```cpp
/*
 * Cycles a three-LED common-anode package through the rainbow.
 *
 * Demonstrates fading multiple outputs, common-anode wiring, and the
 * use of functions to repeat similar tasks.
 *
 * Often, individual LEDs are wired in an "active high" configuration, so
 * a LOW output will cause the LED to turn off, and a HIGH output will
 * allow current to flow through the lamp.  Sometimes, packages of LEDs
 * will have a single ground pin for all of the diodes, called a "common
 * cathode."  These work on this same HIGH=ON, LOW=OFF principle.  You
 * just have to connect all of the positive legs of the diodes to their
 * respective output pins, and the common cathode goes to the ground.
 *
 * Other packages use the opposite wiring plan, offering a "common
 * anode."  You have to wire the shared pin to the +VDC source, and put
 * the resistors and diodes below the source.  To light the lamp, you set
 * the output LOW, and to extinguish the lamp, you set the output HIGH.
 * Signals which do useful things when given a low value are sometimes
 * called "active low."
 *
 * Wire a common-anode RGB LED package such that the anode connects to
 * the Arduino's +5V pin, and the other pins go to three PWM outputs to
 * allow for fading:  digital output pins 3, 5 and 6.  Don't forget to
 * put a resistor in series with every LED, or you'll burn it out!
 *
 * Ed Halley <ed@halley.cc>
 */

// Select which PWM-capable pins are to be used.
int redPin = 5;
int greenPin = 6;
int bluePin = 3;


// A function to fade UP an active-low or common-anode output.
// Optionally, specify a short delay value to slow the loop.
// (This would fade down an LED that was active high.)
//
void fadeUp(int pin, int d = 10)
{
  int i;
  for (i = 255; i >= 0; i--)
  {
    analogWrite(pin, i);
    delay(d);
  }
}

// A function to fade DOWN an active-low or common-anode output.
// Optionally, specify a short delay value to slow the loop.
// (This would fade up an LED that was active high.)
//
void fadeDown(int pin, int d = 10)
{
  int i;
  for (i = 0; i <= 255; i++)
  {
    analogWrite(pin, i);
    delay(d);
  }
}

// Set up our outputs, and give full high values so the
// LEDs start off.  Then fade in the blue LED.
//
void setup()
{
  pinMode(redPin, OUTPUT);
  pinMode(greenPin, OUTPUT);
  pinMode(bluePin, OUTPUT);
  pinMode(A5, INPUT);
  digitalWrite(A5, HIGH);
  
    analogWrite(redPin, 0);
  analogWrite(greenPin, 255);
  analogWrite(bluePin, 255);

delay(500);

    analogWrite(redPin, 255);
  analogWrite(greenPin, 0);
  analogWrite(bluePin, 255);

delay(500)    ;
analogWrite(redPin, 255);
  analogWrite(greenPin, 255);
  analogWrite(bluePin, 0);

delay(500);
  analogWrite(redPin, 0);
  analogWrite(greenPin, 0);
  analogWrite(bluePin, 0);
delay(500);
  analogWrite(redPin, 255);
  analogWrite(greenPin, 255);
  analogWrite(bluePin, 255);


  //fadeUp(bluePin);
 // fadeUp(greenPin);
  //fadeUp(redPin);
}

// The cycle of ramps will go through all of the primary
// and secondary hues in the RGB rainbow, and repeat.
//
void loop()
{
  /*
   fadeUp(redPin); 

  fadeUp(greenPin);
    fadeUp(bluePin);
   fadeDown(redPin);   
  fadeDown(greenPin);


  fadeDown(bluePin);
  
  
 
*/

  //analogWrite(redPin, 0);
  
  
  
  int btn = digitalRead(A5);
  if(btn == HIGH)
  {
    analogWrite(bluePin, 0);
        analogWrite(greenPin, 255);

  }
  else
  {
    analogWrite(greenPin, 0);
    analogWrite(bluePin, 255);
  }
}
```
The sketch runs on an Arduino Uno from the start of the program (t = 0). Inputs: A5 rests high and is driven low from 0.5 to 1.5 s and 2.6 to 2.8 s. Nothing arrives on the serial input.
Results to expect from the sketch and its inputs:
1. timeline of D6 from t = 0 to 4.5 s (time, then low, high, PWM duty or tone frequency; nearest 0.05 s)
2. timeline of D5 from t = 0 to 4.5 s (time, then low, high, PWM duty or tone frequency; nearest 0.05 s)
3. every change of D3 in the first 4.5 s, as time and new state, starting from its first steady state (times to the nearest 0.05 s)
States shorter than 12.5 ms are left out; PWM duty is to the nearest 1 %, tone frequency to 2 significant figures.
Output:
0 s high; 0.5 s low; 1 s high; 1.5 s low; 2 s high; 2.6 s low; 2.8 s high
0 s low; 0.5 s high; 1.5 s low; 2 s high
0 s high; 1 s low; 2.6 s high; 2.8 s low
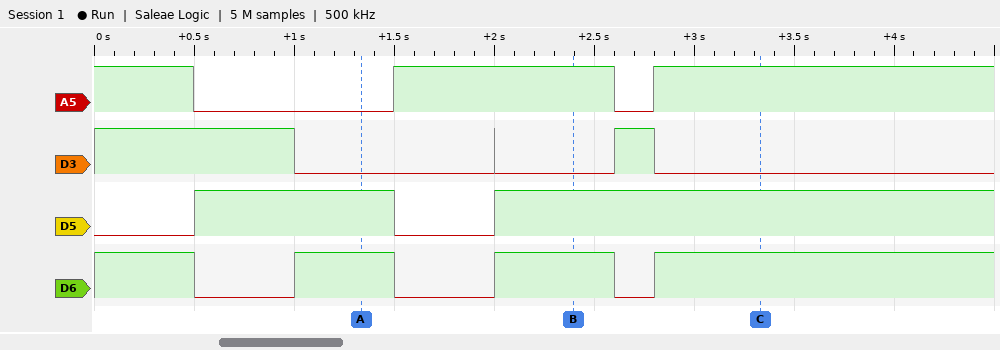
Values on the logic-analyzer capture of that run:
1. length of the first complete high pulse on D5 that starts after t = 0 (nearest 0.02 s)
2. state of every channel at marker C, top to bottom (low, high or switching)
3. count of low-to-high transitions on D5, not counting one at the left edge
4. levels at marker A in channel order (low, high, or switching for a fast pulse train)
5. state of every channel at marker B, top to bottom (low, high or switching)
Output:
1.00 s
A5 high, D3 low, D5 high, D6 high
2
A5 low, D3 low, D5 high, D6 high
A5 high, D3 low, D5 high, D6 high
